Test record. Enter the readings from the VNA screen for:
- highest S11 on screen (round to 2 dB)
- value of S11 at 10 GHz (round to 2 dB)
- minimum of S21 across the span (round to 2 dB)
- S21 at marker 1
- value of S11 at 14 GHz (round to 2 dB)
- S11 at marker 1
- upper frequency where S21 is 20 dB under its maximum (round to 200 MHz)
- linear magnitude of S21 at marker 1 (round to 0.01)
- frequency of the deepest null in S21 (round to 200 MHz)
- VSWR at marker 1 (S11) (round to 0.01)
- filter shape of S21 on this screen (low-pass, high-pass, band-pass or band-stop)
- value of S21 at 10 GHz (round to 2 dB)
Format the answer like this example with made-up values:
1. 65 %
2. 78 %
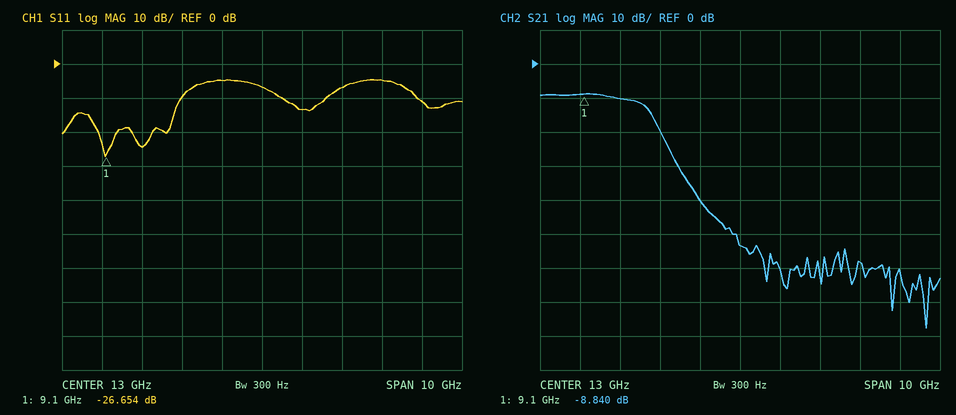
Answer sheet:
1. -4 dB
2. -24 dB
3. -78 dB
4. -8.840 dB
5. -14 dB
6. -26.654 dB
7. 11.4 GHz
8. 0.36
9. 17.6 GHz
10. 1.10
11. low-pass
12. -10 dB
